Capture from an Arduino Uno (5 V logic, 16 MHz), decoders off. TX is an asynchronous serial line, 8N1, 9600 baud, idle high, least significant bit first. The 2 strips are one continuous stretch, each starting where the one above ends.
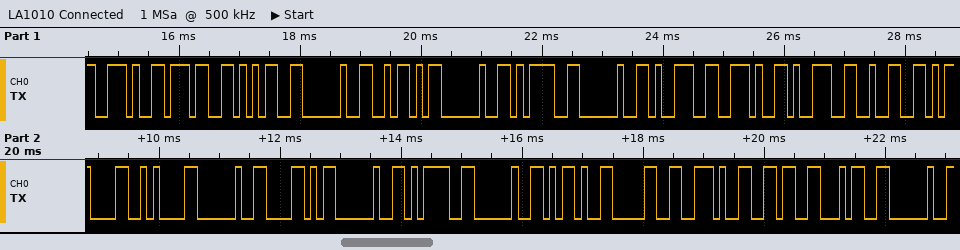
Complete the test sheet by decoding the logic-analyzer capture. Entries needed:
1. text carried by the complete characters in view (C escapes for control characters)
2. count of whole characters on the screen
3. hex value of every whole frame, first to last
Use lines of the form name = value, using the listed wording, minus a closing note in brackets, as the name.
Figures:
text carried by the complete characters in view = ".75 Z = 9.92\r\n X = -0.64 "
count of whole characters on the screen = 25
hex value of every whole frame, first to last = 2E 37 35 20 5A 20 3D 20 39 2E 39 32 0D 0A 20 58 20 3D 20 2D 30 2E 36 34 20
